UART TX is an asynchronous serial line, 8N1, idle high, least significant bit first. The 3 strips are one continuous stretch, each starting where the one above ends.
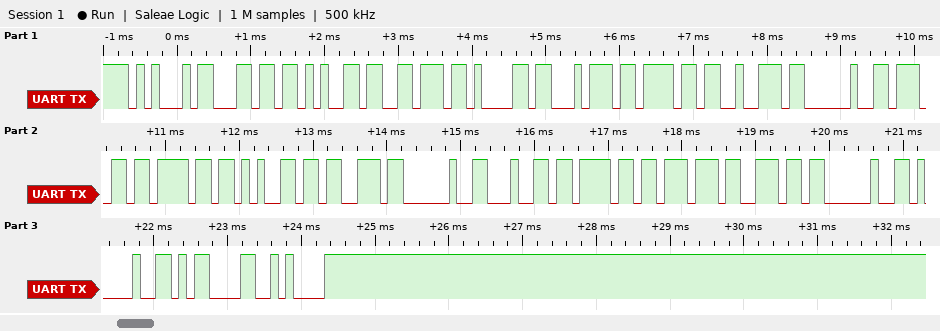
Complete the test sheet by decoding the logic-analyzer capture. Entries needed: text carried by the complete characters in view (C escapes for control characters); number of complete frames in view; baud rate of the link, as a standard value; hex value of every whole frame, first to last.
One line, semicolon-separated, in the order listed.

"Elevator goes down !\r\n"; 22; 9600 baud; 0x45 0x6C 0x65 0x76 0x61 0x74 0x6F 0x72 0x20 0x67 0x6F 0x65 0x73 0x20 0x64 0x6F 0x77 0x6E 0x20 0x21 0x0D 0x0A
